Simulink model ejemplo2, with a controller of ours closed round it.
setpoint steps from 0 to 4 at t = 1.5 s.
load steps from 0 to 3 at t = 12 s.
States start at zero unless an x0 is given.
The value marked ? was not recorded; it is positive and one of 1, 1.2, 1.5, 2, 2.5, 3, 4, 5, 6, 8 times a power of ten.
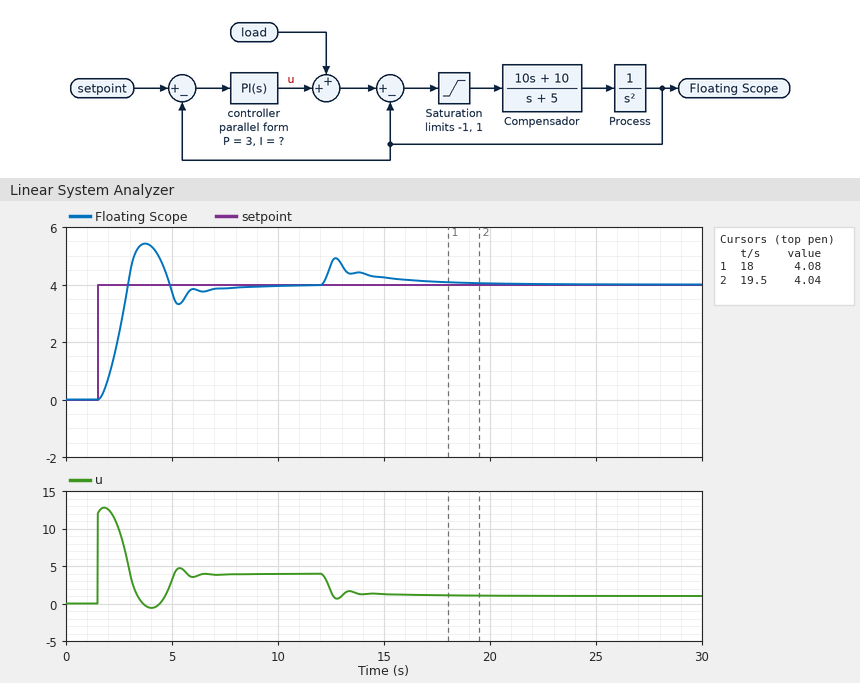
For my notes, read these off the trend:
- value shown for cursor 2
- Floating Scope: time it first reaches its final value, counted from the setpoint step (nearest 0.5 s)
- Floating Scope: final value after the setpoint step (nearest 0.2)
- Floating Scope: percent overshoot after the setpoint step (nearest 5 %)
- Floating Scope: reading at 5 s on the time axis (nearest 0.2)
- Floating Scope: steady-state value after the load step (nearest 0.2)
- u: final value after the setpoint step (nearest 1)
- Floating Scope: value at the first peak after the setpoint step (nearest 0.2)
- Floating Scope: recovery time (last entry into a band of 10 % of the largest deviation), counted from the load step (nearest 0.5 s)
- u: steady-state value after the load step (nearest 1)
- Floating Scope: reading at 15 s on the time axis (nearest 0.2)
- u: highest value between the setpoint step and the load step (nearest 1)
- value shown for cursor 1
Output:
4.04
1.5 s
4.0
35 %
3.8
4.0
4
5.4
5.5 s
1
4.2
13
4.08
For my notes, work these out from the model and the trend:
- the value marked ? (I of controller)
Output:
1.5
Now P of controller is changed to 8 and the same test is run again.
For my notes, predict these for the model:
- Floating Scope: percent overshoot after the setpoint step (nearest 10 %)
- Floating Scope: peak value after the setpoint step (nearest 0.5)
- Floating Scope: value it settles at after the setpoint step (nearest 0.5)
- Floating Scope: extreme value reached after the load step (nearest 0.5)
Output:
30 %
5.0
4.0
4.5
